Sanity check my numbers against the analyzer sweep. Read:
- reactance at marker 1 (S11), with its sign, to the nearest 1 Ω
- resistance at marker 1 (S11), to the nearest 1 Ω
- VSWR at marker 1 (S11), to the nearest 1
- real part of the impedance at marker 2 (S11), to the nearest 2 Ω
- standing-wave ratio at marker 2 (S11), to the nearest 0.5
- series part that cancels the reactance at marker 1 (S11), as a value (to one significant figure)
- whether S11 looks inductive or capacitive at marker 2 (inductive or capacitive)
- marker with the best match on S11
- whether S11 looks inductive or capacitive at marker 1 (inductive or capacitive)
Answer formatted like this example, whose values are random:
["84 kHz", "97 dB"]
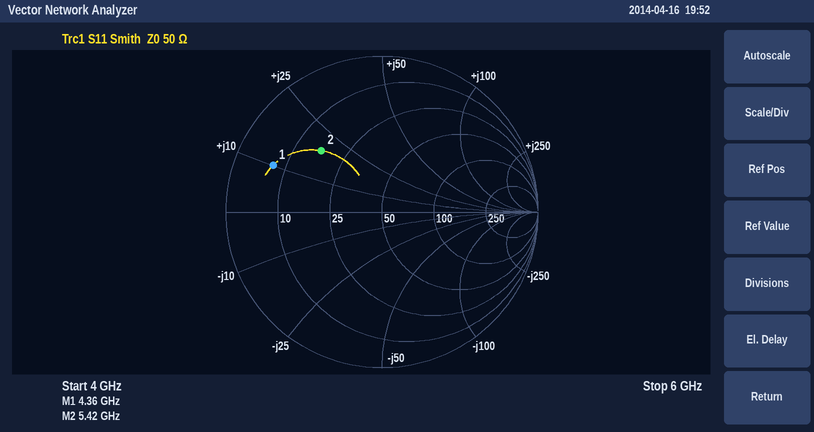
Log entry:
["+10 Ω", "7 Ω", "7", "16 Ω", "3.5", "4 pF", "inductive", "marker 2", "inductive"]
